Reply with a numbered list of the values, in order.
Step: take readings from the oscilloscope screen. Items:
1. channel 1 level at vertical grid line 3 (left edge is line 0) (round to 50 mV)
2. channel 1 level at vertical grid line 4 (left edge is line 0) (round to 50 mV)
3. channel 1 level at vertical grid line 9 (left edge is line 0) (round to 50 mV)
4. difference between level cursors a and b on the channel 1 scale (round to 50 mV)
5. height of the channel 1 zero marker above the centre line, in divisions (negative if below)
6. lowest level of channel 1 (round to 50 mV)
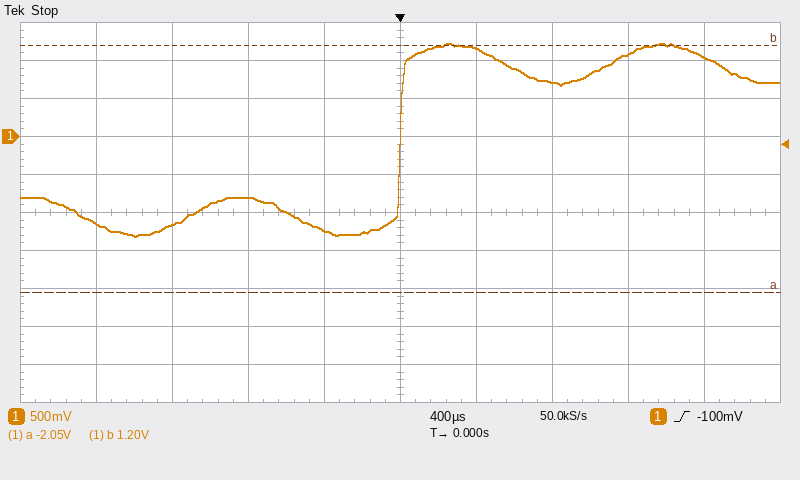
1. -800 mV
2. -1.25 V
3. 1.05 V
4. 3.25 V
5. +2.0 div
6. -1.30 V
